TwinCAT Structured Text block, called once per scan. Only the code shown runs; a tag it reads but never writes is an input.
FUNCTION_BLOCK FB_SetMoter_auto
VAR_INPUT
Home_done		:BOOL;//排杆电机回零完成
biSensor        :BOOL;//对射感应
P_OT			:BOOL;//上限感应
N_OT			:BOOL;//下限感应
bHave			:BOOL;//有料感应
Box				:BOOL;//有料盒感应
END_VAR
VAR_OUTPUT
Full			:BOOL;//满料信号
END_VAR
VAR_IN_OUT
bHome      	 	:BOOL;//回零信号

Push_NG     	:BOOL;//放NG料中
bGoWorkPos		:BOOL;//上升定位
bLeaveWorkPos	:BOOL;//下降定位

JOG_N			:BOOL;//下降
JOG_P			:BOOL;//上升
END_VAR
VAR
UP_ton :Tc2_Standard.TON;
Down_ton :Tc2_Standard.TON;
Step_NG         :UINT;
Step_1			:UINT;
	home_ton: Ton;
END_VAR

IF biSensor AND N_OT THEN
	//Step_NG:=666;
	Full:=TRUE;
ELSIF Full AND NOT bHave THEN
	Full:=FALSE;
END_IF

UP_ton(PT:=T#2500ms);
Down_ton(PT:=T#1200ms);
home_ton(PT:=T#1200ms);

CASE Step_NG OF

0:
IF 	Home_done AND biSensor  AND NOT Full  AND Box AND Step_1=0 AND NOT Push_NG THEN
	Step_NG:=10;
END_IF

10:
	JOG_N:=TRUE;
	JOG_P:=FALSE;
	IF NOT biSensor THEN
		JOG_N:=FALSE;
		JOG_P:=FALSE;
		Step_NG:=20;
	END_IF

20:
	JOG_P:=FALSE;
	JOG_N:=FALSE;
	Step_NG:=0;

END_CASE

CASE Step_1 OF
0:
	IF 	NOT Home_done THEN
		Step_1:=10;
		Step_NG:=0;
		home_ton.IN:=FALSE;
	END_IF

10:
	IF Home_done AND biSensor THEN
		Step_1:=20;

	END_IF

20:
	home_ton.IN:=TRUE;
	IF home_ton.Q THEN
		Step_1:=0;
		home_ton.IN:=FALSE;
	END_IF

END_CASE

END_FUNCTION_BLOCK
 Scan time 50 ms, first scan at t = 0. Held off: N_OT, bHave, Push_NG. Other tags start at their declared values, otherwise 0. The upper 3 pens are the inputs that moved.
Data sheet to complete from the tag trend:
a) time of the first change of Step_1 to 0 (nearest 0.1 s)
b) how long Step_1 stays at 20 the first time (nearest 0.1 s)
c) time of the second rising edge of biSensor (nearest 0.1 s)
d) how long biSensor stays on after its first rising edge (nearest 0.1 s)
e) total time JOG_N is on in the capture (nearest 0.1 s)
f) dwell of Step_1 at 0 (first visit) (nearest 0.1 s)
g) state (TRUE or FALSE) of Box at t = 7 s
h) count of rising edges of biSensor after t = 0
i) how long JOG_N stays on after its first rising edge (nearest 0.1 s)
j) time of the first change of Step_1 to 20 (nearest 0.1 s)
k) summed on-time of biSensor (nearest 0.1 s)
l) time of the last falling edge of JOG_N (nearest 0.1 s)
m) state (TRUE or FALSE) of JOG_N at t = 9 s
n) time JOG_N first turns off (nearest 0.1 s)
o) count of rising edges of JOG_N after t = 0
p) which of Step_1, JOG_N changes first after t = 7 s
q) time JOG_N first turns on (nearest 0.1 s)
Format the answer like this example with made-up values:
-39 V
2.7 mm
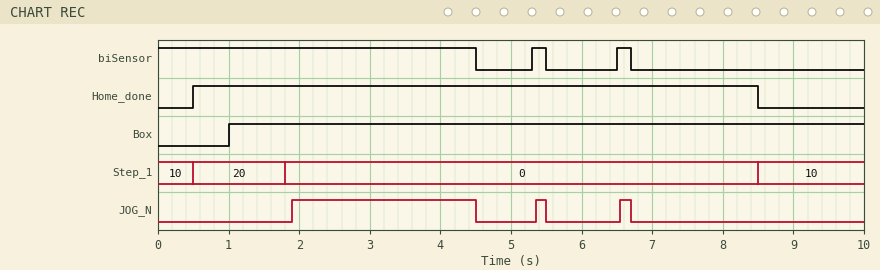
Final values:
1.8 s
1.3 s
6.5 s
0.2 s
2.9 s
6.7 s
TRUE
2
2.6 s
0.5 s
4.9 s
6.7 s
FALSE
4.5 s
3
Step_1
1.9 s
